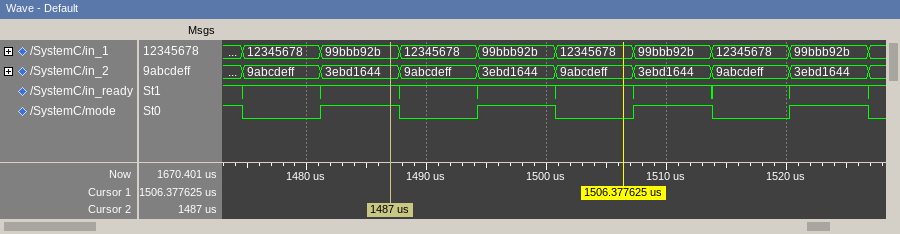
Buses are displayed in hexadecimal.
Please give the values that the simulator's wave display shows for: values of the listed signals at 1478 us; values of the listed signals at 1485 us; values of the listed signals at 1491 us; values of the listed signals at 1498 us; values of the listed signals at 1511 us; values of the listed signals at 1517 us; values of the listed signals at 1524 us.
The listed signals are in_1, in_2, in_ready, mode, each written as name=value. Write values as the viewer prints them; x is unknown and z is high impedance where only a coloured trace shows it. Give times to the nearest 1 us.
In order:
in_1=12345678, in_2=9abcdeff, in_ready=1, mode=0
in_1=99bbb92b, in_2=3ebd1644, in_ready=1, mode=1
in_1=12345678, in_2=9abcdeff, in_ready=1, mode=0
in_1=99bbb92b, in_2=3ebd1644, in_ready=1, mode=1
in_1=99bbb92b, in_2=3ebd1644, in_ready=1, mode=1
in_1=12345678, in_2=9abcdeff, in_ready=1, mode=0
in_1=99bbb92b, in_2=3ebd1644, in_ready=1, mode=1
